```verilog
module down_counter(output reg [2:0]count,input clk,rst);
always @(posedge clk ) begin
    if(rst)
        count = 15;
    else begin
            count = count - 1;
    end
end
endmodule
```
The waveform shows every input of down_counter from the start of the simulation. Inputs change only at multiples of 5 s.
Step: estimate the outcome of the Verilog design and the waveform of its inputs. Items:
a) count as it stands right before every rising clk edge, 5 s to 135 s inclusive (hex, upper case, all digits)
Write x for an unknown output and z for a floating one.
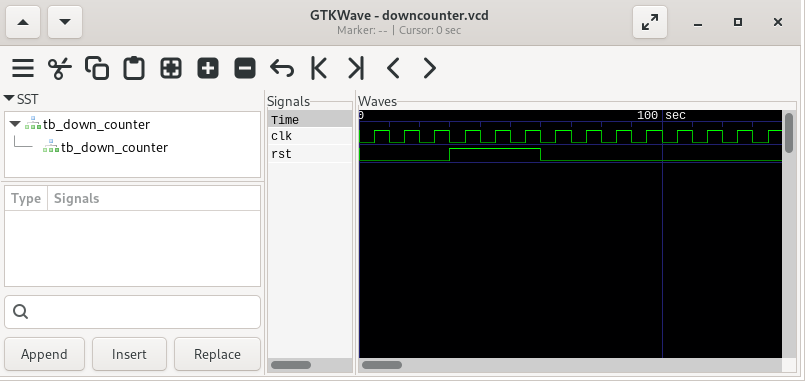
x, x, x, x, 7, 7, 7, 6, 5, 4, 3, 2, 1, 0
